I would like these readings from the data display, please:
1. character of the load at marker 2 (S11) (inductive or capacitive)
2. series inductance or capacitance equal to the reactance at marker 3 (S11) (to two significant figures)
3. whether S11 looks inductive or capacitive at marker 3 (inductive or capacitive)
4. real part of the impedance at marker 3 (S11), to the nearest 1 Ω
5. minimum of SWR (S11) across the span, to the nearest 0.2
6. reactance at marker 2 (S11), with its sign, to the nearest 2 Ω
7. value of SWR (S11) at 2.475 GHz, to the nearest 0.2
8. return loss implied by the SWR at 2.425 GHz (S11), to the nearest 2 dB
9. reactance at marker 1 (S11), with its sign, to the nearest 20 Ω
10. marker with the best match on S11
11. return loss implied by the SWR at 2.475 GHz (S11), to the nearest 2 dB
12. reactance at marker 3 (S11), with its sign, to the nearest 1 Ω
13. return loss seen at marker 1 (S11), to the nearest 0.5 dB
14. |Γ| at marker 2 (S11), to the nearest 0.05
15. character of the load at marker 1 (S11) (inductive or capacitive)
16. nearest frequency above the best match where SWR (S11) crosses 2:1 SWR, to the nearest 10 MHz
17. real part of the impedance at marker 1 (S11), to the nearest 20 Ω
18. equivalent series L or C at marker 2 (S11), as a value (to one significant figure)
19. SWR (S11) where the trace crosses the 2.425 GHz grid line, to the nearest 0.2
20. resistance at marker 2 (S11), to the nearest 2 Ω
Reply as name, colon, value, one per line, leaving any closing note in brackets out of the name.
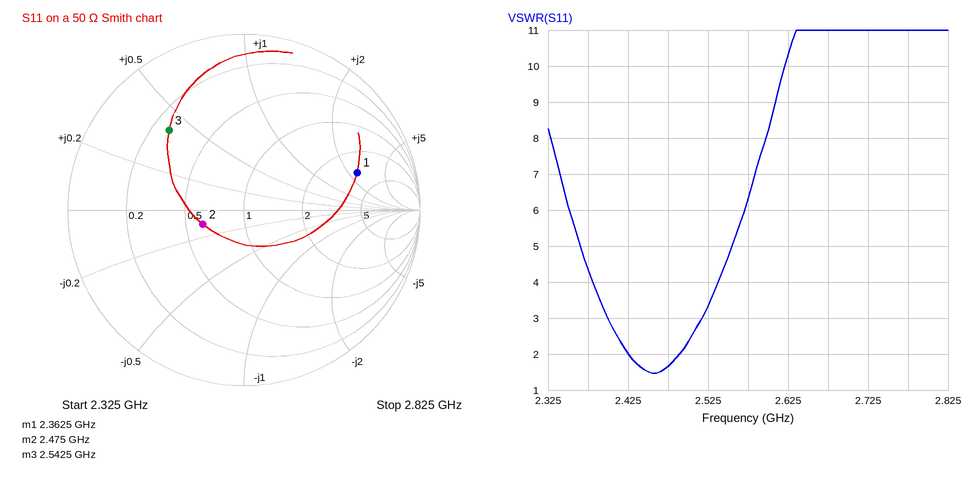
character of the load at marker 2 (S11): capacitive
series inductance or capacitance equal to the reactance at marker 3 (S11): 1.3 nH
whether S11 looks inductive or capacitive at marker 3: inductive
real part of the impedance at marker 3 (S11), to the nearest 1 Ω: 14 Ω
minimum of SWR (S11) across the span, to the nearest 0.2: 1.4
reactance at marker 2 (S11), with its sign, to the nearest 2 Ω: -6 Ω
value of SWR (S11) at 2.475 GHz, to the nearest 0.2: 1.6
return loss implied by the SWR at 2.425 GHz (S11), to the nearest 2 dB: 10 dB
reactance at marker 1 (S11), with its sign, to the nearest 20 Ω: +120 Ω
marker with the best match on S11: marker 2
return loss implied by the SWR at 2.475 GHz (S11), to the nearest 2 dB: 12 dB
reactance at marker 3 (S11), with its sign, to the nearest 1 Ω: +20 Ω
return loss seen at marker 1 (S11), to the nearest 0.5 dB: 3.5 dB
|Γ| at marker 2 (S11), to the nearest 0.05: 0.25
character of the load at marker 1 (S11): inductive
nearest frequency above the best match where SWR (S11) crosses 2:1 SWR, to the nearest 10 MHz: 2.49 GHz
real part of the impedance at marker 1 (S11), to the nearest 20 Ω: 160 Ω
equivalent series L or C at marker 2 (S11), as a value: 10 pF
SWR (S11) where the trace crosses the 2.425 GHz grid line, to the nearest 0.2: 2.0
resistance at marker 2 (S11), to the nearest 2 Ω: 30 Ω
